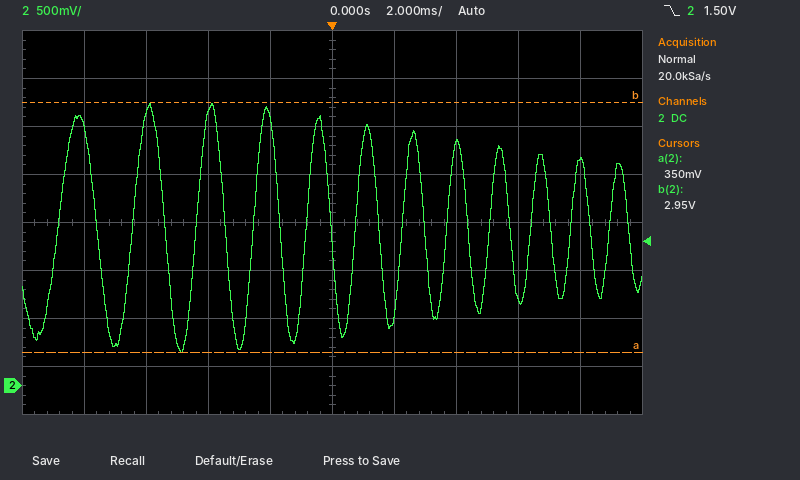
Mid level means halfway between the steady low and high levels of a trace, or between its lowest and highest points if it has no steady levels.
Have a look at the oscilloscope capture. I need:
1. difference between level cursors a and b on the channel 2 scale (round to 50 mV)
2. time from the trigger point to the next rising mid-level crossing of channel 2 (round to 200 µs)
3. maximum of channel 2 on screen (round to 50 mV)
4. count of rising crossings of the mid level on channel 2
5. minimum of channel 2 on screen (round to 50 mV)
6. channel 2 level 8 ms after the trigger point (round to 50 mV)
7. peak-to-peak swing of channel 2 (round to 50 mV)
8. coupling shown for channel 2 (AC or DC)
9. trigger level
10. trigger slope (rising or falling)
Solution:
2.60 V
800 µs
2.95 V
12
350 mV
2.35 V
2.60 V
DC
1.50 V
falling
